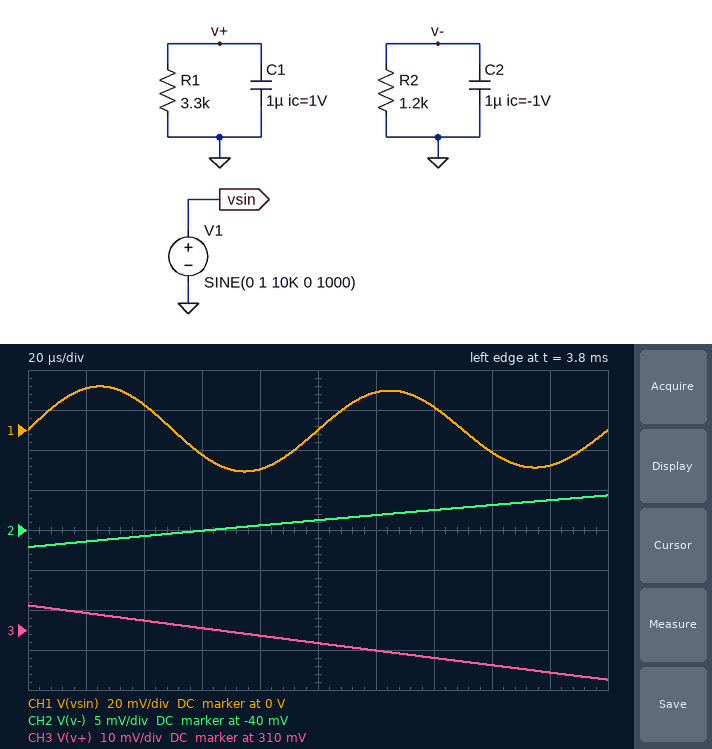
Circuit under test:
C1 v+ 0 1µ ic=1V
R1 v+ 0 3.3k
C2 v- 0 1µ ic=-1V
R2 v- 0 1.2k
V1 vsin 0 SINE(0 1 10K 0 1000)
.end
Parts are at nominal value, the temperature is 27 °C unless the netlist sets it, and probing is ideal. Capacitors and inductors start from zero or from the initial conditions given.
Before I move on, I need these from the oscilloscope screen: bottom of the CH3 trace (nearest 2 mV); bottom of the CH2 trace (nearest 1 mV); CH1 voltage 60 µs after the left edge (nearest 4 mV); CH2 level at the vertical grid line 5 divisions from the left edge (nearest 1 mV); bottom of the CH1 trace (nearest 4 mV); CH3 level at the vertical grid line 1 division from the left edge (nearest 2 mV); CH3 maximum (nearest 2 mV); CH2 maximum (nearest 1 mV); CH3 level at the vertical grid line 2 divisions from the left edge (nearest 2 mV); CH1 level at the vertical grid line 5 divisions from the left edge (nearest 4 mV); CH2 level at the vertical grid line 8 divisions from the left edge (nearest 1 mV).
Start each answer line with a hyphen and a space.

- 298 mV
- -42 mV
- -12 mV
- -39 mV
- -20 mV
- 314 mV
- 316 mV
- -36 mV
- 312 mV
- 0 V
- -37 mV
